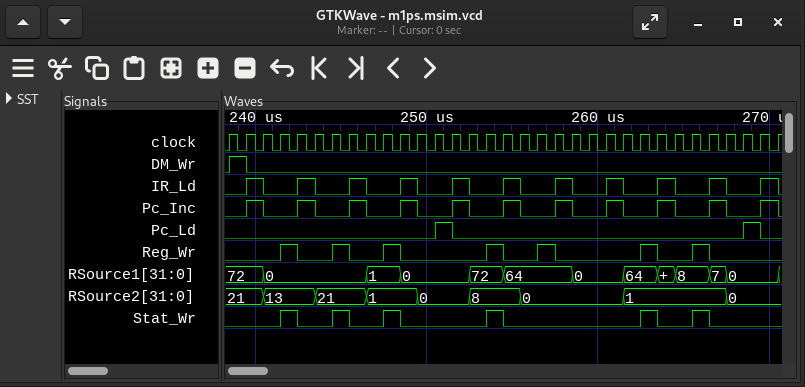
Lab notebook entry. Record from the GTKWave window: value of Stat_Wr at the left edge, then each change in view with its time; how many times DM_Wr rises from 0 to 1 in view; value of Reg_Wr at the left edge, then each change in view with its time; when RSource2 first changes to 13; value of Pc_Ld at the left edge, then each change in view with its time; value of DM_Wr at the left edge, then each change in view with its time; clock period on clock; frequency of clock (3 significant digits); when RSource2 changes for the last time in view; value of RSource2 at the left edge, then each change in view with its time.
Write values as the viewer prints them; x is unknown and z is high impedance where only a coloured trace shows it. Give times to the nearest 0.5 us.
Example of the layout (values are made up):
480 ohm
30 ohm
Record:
0, 1 at 241.5 us, 0 at 242.5 us, 1 at 244.5 us, 0 at 245.5 us, 1 at 247.5 us, 0 at 248.5 us, 1 at 253.5 us, 0 at 254.5 us, 1 at 262.5 us, 0 at 263.5 us, 1 at 265.5 us, 0 at 266.5 us
1
0, 1 at 241.5 us, 0 at 242.5 us, 1 at 244.5 us, 0 at 245.5 us, 1 at 247.5 us, 0 at 248.5 us, 1 at 253.5 us, 0 at 254.5 us, 1 at 256.5 us, 0 at 257.5 us, 1 at 262.5 us, 0 at 263.5 us, 1 at 265.5 us, 0 at 266.5 us
240.5 us
0, 1 at 250.5 us, 0 at 251.5 us, 1 at 268.5 us, 0 at 269.5 us
0, 1 at 238.5 us, 0 at 239.5 us
1 us
1.00 MHz
267.5 us
21, 13 at 240.5 us, 21 at 243.5 us, 1 at 246.5 us, 0 at 249.5 us, 8 at 252.5 us, 0 at 255.5 us, 1 at 261.5 us, 0 at 267.5 us
